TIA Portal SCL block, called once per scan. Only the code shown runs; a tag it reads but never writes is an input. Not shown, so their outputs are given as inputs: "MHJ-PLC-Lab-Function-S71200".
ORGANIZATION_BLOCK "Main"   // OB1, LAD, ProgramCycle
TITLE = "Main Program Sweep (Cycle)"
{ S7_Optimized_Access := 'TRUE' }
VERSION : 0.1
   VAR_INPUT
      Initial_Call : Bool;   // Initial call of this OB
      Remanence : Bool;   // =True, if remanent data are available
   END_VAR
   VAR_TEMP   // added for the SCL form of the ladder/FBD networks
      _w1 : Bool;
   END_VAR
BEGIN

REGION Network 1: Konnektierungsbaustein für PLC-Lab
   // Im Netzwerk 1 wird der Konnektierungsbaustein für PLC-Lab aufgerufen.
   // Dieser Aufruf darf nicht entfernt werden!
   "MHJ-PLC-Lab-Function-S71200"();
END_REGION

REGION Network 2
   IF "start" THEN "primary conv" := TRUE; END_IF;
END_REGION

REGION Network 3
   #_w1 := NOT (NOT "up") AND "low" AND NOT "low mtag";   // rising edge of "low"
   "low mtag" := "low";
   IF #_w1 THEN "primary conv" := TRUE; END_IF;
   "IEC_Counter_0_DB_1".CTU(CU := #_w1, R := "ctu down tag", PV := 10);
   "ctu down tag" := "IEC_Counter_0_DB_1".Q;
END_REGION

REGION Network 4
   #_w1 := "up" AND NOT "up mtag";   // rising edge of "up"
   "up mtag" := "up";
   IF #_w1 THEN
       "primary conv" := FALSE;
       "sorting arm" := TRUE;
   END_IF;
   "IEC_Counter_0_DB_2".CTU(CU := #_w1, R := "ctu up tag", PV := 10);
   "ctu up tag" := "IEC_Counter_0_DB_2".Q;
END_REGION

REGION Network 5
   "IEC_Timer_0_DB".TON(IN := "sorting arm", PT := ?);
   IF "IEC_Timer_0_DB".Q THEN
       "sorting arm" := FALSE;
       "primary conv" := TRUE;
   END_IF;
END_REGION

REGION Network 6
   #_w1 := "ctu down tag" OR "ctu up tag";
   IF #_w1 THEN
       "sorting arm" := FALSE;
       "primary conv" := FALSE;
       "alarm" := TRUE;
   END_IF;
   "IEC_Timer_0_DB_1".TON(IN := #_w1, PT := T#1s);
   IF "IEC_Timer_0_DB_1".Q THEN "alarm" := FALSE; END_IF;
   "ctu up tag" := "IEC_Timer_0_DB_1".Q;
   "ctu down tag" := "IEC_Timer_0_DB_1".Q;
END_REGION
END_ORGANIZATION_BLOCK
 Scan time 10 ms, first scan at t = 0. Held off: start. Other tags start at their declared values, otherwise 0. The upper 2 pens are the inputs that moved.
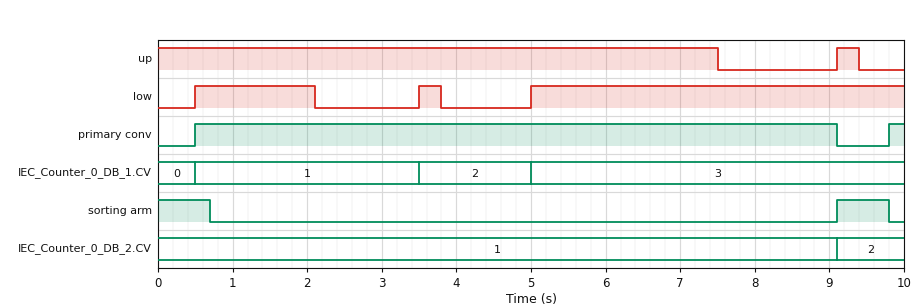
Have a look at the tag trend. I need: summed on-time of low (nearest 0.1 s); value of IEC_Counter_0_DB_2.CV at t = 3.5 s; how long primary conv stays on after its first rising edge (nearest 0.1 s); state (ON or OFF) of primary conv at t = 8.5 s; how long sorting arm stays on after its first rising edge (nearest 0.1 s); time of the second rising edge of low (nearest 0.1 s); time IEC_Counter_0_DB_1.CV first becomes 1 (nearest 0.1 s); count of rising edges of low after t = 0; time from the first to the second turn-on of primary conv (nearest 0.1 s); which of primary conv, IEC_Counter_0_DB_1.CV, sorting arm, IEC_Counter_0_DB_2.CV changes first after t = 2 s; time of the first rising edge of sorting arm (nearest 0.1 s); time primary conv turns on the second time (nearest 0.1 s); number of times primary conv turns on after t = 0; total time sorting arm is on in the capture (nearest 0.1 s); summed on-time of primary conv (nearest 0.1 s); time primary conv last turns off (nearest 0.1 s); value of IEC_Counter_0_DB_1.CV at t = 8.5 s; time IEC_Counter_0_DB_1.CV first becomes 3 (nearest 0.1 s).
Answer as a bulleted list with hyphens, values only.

- 6.9 s
- 1
- 8.6 s
- ON
- 0.7 s
- 3.5 s
- 0.5 s
- 3
- 9.3 s
- IEC_Counter_0_DB_1.CV
- 9.1 s
- 9.8 s
- 2
- 1.4 s
- 8.8 s
- 9.1 s
- 3
- 5.0 s
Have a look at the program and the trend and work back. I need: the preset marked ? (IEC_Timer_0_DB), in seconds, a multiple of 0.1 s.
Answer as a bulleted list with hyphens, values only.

- 0.7 s
